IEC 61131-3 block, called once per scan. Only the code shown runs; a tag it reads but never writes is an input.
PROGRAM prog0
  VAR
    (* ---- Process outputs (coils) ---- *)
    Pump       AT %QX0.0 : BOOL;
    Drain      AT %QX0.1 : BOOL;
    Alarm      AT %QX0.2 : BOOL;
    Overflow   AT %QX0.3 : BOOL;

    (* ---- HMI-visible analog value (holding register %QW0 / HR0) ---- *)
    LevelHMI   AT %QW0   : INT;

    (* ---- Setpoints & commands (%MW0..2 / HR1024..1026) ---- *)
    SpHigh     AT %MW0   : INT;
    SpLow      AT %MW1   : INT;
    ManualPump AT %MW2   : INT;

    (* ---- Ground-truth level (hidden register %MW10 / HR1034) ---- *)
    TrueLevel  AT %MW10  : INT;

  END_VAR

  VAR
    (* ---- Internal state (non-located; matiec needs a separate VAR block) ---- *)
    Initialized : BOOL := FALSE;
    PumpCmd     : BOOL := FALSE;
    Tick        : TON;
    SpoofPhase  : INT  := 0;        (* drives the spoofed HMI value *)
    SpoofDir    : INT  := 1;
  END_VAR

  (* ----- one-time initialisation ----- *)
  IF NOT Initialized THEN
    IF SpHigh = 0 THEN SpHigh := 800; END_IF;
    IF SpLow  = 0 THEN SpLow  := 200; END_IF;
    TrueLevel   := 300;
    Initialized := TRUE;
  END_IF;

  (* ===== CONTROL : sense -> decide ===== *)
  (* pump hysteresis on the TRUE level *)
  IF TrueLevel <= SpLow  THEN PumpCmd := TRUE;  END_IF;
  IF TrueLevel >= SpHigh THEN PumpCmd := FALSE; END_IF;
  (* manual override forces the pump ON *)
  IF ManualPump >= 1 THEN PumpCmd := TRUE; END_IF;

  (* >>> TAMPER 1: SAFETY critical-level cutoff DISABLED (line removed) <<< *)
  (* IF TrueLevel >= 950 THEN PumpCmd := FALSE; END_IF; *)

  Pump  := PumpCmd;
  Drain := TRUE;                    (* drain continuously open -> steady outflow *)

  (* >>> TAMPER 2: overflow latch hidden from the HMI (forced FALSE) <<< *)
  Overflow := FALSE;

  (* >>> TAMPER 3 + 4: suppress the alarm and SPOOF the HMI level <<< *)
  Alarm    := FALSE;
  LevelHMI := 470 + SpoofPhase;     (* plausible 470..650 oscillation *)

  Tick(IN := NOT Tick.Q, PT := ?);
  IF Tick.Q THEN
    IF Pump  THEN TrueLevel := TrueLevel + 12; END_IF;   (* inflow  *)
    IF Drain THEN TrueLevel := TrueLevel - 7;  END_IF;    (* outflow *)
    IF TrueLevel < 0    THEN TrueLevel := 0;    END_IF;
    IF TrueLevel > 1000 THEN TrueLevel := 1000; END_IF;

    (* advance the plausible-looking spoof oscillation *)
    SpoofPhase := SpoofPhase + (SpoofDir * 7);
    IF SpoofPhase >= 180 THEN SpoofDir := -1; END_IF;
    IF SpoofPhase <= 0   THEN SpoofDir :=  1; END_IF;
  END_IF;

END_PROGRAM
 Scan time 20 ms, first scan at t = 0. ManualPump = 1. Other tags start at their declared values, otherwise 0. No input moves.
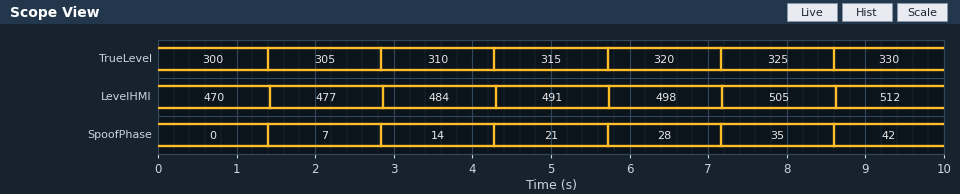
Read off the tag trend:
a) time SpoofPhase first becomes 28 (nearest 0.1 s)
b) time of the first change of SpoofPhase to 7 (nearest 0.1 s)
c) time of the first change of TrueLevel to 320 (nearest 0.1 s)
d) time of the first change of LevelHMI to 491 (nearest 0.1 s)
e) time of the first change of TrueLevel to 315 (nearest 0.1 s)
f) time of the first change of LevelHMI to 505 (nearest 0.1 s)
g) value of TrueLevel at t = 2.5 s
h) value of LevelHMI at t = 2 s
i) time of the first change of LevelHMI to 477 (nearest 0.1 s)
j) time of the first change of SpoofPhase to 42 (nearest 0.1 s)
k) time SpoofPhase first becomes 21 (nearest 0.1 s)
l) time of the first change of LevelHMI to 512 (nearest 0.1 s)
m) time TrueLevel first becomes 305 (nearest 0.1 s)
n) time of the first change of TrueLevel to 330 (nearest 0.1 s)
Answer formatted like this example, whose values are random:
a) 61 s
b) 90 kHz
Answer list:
a) 5.7 s
b) 1.4 s
c) 5.7 s
d) 4.3 s
e) 4.3 s
f) 7.2 s
g) 305
h) 477
i) 1.4 s
j) 8.6 s
k) 4.3 s
l) 8.6 s
m) 1.4 s
n) 8.6 s
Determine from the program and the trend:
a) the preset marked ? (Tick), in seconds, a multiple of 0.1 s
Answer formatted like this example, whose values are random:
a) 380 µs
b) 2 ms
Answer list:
a) 1.4 s
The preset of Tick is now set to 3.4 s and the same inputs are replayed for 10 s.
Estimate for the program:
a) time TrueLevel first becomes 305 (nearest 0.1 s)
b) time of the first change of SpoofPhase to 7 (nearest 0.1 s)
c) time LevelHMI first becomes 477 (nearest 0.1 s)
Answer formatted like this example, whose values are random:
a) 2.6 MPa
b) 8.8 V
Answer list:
a) 3.4 s
b) 3.4 s
c) 3.4 s
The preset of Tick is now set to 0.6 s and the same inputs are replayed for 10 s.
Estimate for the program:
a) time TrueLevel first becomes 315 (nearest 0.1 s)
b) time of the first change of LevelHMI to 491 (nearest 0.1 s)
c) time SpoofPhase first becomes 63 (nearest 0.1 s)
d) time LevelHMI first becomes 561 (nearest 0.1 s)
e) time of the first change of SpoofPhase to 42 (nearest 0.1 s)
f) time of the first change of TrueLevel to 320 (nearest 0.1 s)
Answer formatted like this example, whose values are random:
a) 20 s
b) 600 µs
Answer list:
a) 1.9 s
b) 1.9 s
c) 5.7 s
d) 8.3 s
e) 3.8 s
f) 2.5 s
